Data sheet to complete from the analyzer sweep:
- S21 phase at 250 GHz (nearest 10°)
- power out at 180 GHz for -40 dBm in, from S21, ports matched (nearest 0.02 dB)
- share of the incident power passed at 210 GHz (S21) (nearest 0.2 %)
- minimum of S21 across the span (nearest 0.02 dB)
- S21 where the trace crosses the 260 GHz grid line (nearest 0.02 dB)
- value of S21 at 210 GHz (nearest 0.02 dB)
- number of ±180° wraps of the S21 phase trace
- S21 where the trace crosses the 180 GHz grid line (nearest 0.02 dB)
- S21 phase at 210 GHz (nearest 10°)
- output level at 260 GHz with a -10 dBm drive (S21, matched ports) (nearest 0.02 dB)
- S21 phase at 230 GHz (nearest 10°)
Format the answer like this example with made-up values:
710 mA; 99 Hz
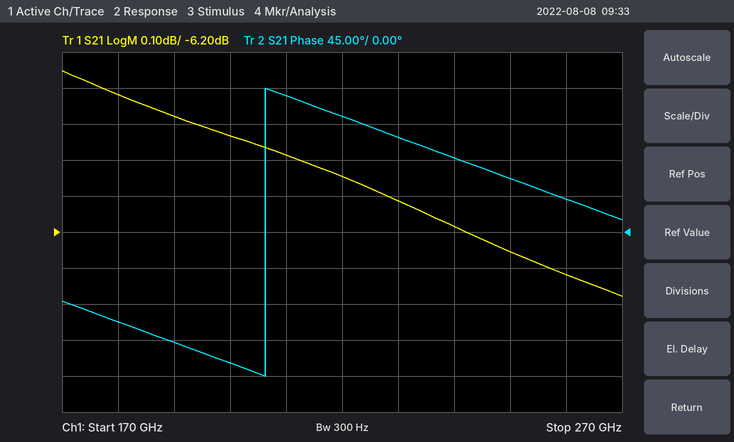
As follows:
70°; -45.82 dBm; 25.2 %; -6.38 dB; -6.32 dB; -5.98 dB; 1; -5.82 dB; 170°; -16.32 dBm; 120°
